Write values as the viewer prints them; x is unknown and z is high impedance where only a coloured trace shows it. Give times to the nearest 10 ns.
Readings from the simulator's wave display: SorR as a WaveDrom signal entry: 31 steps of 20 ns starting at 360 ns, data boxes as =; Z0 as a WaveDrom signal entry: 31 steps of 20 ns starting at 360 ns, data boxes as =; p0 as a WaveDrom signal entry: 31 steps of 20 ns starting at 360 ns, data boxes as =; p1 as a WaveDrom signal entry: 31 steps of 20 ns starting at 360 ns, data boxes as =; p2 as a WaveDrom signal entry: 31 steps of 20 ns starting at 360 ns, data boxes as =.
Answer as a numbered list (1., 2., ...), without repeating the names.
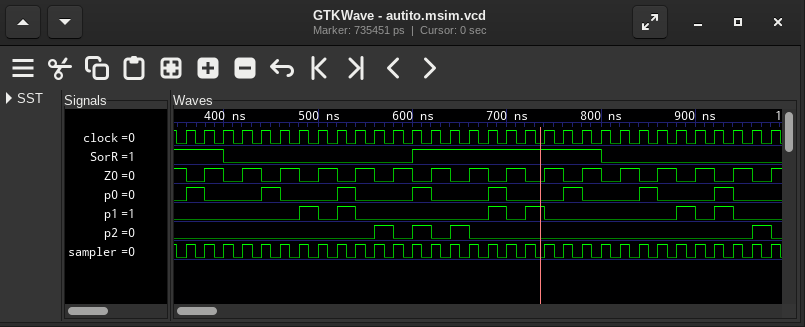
1. {name: 'SorR', wave: '1.0.........1.........0........'}
2. {name: 'Z0', wave: '0101010101010101010101010101010'}
3. {name: 'p0', wave: '10..10..10..10..10..10..10..10.'}
4. {name: 'p1', wave: '0.....1010......1010......1010.'}
5. {name: 'p2', wave: '0.........101010..............1'}
